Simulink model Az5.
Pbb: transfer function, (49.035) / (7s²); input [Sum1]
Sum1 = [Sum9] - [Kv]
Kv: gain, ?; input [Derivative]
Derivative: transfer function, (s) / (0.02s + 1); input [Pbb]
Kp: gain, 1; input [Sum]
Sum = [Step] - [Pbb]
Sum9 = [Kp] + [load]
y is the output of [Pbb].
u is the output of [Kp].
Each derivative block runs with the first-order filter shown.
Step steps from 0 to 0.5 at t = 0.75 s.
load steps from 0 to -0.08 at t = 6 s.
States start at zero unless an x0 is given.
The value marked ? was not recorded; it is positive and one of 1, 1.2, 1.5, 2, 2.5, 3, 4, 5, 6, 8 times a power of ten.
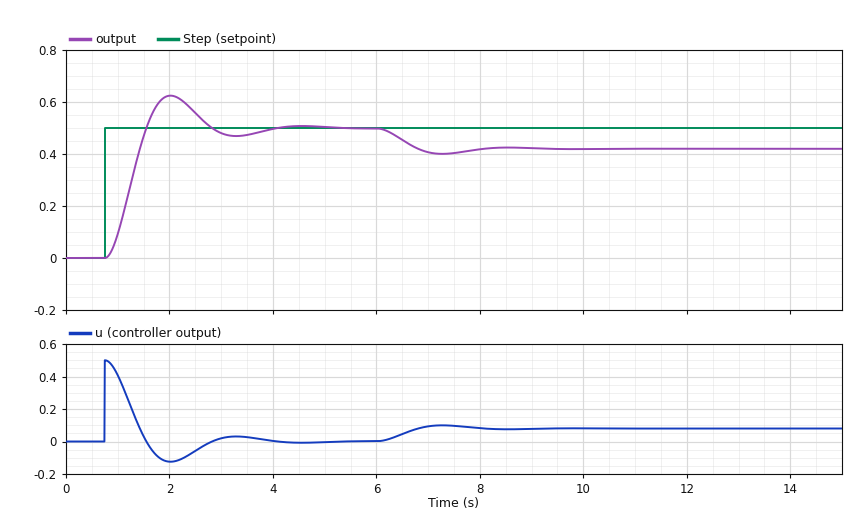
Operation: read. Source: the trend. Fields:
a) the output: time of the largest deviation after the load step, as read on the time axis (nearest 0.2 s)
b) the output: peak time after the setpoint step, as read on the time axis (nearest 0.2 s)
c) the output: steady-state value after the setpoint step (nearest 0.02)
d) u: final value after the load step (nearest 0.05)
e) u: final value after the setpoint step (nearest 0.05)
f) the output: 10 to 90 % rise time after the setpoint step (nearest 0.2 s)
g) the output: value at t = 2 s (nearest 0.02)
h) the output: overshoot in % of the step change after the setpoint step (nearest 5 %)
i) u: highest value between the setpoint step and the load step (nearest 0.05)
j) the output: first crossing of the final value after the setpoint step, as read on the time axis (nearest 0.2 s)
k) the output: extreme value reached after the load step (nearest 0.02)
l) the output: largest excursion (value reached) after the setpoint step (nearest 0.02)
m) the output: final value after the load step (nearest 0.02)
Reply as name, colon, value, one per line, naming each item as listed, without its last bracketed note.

the output: time of the largest deviation after the load step, as read on the time axis: 7.2 s
the output: peak time after the setpoint step, as read on the time axis: 2.0 s
the output: steady-state value after the setpoint step: 0.50
u: final value after the load step: 0.10
u: final value after the setpoint step: 0.00
the output: 10 to 90 % rise time after the setpoint step: 0.6 s
the output: value at t = 2 s: 0.62
the output: overshoot in % of the step change after the setpoint step: 25 %
u: highest value between the setpoint step and the load step: 0.50
the output: first crossing of the final value after the setpoint step, as read on the time axis: 1.6 s
the output: extreme value reached after the load step: 0.40
the output: largest excursion (value reached) after the setpoint step: 0.62
the output: final value after the load step: 0.42
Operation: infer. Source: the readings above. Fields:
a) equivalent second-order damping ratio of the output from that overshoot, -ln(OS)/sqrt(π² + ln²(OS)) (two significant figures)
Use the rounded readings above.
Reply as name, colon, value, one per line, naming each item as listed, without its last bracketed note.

equivalent second-order damping ratio of the output from that overshoot, -ln(OS)/sqrt(π² + ln²(OS)): 0.40
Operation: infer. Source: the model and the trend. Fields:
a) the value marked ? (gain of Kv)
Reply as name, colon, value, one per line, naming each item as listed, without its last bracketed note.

the value marked ?: 0.3
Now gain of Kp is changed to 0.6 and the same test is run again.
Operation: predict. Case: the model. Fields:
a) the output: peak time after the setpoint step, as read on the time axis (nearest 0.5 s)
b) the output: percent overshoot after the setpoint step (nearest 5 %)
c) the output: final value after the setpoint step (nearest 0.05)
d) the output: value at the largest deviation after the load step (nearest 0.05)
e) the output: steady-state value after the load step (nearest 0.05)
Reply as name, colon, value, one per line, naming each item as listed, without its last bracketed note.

the output: peak time after the setpoint step, as read on the time axis: 2.5 s
the output: percent overshoot after the setpoint step: 15 %
the output: final value after the setpoint step: 0.50
the output: value at the largest deviation after the load step: 0.35
the output: steady-state value after the load step: 0.35
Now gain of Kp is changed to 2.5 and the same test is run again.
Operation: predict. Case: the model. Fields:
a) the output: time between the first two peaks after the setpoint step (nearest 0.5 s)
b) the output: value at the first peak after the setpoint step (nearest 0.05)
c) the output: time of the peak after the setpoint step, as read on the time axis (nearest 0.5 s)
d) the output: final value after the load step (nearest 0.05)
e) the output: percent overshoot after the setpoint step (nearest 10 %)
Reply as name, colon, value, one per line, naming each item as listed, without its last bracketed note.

the output: time between the first two peaks after the setpoint step: 1.5 s
the output: value at the first peak after the setpoint step: 0.70
the output: time of the peak after the setpoint step, as read on the time axis: 1.5 s
the output: final value after the load step: 0.45
the output: percent overshoot after the setpoint step: 40 %
